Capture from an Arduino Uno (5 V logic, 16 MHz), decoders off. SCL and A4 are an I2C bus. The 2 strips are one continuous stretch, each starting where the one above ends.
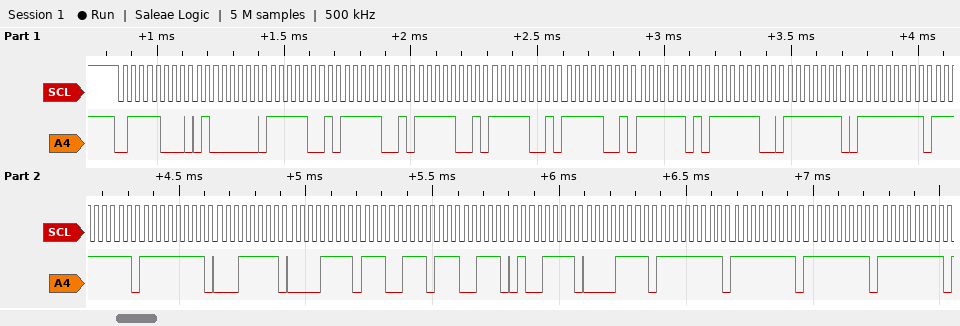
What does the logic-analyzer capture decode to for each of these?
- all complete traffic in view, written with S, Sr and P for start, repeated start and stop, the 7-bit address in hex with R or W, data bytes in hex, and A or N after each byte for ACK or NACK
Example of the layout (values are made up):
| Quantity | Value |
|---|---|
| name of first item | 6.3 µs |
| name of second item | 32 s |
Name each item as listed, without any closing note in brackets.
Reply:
| Quantity | Value |
|---|---|
| all complete traffic in view, written with S, Sr and P for start, repeated start and stop, the 7-bit address in hex with R or W, data bytes in hex, and A or N after each byte for ACK or NACK | S 3CW A 40 A F9 A F9 A F9 A F9 A F9 A FD A FC A FE A FF A FF A FF A 1F A 0F A E7 A E7 A 4F A 0F A FF A FF A FF A FF A |
